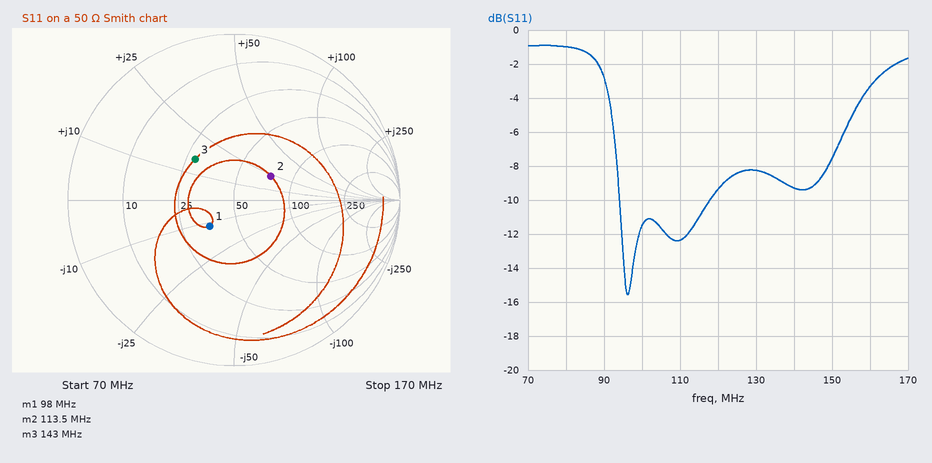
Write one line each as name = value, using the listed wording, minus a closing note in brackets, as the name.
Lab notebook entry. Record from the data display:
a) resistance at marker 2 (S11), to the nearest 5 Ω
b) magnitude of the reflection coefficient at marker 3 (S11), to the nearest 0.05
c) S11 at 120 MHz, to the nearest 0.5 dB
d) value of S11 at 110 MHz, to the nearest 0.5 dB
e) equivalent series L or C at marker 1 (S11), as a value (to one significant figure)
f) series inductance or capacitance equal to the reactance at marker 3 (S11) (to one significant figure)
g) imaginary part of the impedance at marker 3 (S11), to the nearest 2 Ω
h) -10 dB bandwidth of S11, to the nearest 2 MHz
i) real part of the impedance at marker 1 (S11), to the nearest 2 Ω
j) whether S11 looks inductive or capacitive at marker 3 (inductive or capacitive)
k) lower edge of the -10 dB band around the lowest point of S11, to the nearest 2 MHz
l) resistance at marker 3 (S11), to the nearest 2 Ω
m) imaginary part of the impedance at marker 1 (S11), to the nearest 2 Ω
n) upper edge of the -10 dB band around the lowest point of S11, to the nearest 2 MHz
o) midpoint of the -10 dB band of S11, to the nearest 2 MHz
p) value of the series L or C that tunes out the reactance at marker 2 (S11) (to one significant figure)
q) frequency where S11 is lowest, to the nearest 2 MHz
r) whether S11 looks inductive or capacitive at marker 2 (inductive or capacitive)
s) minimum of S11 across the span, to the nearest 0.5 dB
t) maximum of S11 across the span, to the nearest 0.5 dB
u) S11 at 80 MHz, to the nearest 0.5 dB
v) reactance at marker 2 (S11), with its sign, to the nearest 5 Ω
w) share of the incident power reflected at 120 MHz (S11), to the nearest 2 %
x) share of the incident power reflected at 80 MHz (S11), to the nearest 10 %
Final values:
resistance at marker 2 (S11), to the nearest 5 Ω = 75 Ω
magnitude of the reflection coefficient at marker 3 (S11), to the nearest 0.05 = 0.35
S11 at 120 MHz, to the nearest 0.5 dB = -9.5 dB
value of S11 at 110 MHz, to the nearest 0.5 dB = -12.5 dB
equivalent series L or C at marker 1 (S11), as a value = 100 pF
series inductance or capacitance equal to the reactance at marker 3 (S11) = 20 nH
imaginary part of the impedance at marker 3 (S11), to the nearest 2 Ω = +16 Ω
-10 dB bandwidth of S11, to the nearest 2 MHz = 24 MHz
real part of the impedance at marker 1 (S11), to the nearest 2 Ω = 36 Ω
whether S11 looks inductive or capacitive at marker 3 = inductive
lower edge of the -10 dB band around the lowest point of S11, to the nearest 2 MHz = 94 MHz
resistance at marker 3 (S11), to the nearest 2 Ω = 28 Ω
imaginary part of the impedance at marker 1 (S11), to the nearest 2 Ω = -12 Ω
upper edge of the -10 dB band around the lowest point of S11, to the nearest 2 MHz = 118 MHz
midpoint of the -10 dB band of S11, to the nearest 2 MHz = 106 MHz
value of the series L or C that tunes out the reactance at marker 2 (S11) = 60 pF
frequency where S11 is lowest, to the nearest 2 MHz = 96 MHz
whether S11 looks inductive or capacitive at marker 2 = inductive
minimum of S11 across the span, to the nearest 0.5 dB = -15.5 dB
maximum of S11 across the span, to the nearest 0.5 dB = -1.0 dB
S11 at 80 MHz, to the nearest 0.5 dB = -1.0 dB
reactance at marker 2 (S11), with its sign, to the nearest 5 Ω = +25 Ω
share of the incident power reflected at 120 MHz (S11), to the nearest 2 % = 12 %
share of the incident power reflected at 80 MHz (S11), to the nearest 10 % = 80 %
